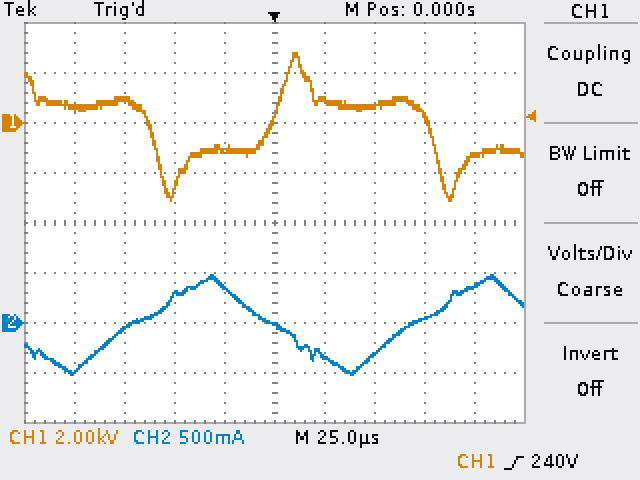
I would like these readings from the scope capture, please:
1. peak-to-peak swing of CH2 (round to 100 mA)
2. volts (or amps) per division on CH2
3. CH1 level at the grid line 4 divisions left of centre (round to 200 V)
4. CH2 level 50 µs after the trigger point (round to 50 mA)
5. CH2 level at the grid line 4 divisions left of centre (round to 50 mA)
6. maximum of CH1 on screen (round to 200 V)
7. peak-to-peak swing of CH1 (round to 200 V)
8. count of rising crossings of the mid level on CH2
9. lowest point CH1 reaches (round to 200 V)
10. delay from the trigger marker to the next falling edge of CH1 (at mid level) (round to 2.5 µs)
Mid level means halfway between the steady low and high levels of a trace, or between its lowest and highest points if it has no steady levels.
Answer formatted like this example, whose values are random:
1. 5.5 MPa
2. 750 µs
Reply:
1. 1.00 A
2. 500 mA
3. 600 V
4. -300 mA
5. -500 mA
6. 2.8 kV
7. 6.0 kV
8. 2
9. -3.2 kV
10. 77.5 µs
